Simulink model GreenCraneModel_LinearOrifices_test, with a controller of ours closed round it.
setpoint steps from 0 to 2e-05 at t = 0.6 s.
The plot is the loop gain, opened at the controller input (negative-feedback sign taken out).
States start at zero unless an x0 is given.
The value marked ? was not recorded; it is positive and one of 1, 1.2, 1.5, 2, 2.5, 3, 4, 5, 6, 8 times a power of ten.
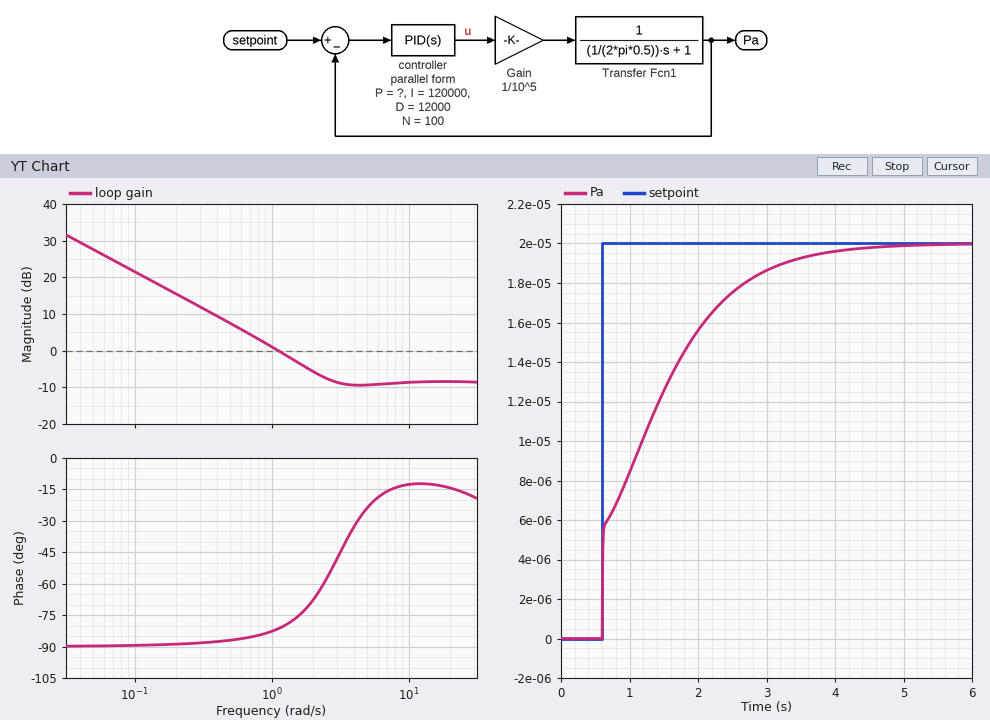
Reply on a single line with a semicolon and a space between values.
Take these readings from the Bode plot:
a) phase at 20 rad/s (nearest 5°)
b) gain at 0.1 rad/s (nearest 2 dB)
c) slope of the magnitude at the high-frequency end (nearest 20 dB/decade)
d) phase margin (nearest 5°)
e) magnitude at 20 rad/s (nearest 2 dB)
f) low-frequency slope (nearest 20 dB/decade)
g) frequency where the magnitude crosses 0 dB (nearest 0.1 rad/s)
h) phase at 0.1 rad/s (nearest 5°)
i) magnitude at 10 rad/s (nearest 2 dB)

-15°; 22 dB; 0 dB/decade; 100°; -8 dB; -20 dB/decade; 1.1 rad/s; -90°; -8 dB
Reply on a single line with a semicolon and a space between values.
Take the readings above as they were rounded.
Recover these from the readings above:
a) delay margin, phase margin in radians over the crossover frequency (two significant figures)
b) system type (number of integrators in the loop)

1.6 s; 1
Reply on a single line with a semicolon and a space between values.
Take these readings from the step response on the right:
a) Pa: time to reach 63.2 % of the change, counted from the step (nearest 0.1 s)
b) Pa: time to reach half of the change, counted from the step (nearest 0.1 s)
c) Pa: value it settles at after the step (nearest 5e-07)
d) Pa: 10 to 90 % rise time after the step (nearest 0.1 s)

0.9 s; 0.6 s; 0.0000200; 2.1 s
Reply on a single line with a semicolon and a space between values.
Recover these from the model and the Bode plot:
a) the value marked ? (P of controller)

50000
